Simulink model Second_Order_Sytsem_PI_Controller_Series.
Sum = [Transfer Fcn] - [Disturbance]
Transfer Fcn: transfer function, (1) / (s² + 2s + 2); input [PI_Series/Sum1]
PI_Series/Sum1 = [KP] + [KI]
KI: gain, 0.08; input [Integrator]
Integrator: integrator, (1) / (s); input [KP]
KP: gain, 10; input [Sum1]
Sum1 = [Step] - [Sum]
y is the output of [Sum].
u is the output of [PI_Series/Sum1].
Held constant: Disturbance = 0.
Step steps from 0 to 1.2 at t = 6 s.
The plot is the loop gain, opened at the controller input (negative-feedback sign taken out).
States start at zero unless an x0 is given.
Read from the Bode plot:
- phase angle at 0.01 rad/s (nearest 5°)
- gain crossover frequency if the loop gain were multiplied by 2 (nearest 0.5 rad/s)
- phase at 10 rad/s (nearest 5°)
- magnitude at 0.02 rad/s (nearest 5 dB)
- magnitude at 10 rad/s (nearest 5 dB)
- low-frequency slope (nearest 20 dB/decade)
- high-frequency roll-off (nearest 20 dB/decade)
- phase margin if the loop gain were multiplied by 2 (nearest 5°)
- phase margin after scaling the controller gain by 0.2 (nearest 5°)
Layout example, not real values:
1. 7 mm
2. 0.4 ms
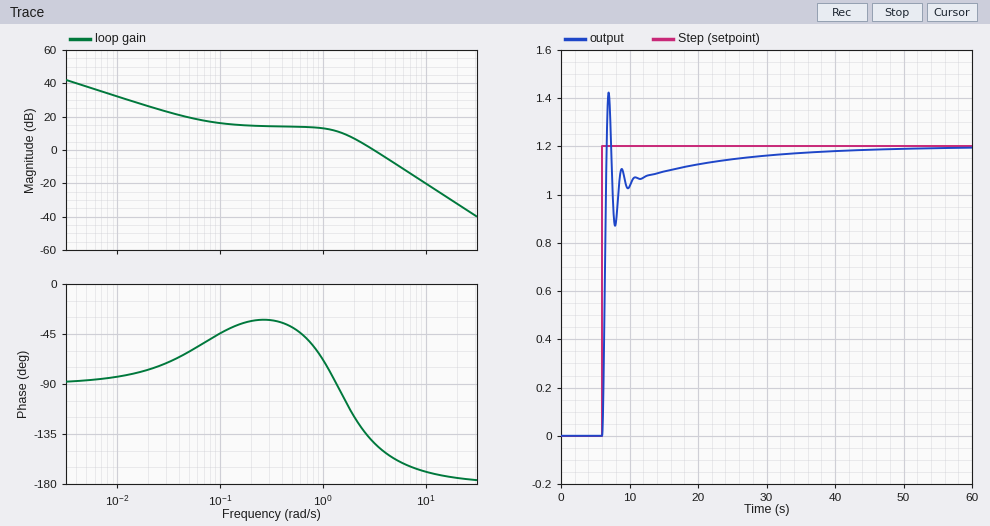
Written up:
1. -85°
2. 4.5 rad/s
3. -170°
4. 25 dB
5. -20 dB
6. -20 dB/decade
7. -40 dB/decade
8. 25°
9. 140°
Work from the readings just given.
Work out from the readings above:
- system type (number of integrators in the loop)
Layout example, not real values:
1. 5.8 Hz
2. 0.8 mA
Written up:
1. 1
